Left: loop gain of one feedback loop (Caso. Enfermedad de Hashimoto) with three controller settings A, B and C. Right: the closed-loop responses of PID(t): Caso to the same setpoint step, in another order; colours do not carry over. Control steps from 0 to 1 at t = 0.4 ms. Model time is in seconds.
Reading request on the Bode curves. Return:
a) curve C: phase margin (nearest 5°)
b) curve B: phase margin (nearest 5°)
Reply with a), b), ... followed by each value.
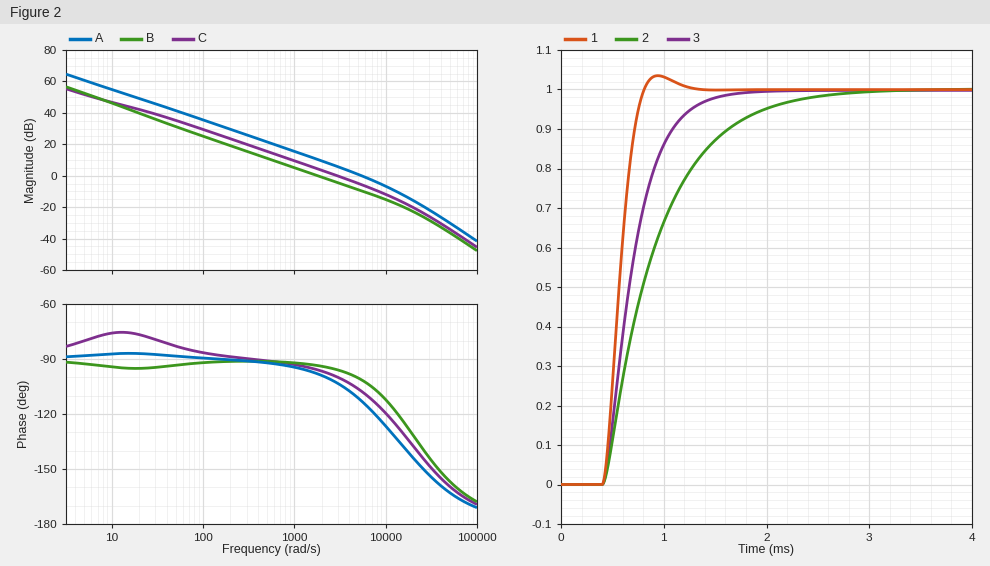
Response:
a) 80°
b) 85°
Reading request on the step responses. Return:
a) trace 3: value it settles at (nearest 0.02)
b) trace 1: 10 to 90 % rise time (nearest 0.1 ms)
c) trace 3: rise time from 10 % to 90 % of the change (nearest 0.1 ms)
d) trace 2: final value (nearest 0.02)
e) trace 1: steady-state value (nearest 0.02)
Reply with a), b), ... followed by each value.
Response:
a) 1.00
b) 0.3 ms
c) 0.6 ms
d) 1.00
e) 1.00
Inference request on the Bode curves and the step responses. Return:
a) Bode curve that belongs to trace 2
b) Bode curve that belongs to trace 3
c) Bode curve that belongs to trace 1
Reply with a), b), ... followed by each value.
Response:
a) B
b) C
c) A
